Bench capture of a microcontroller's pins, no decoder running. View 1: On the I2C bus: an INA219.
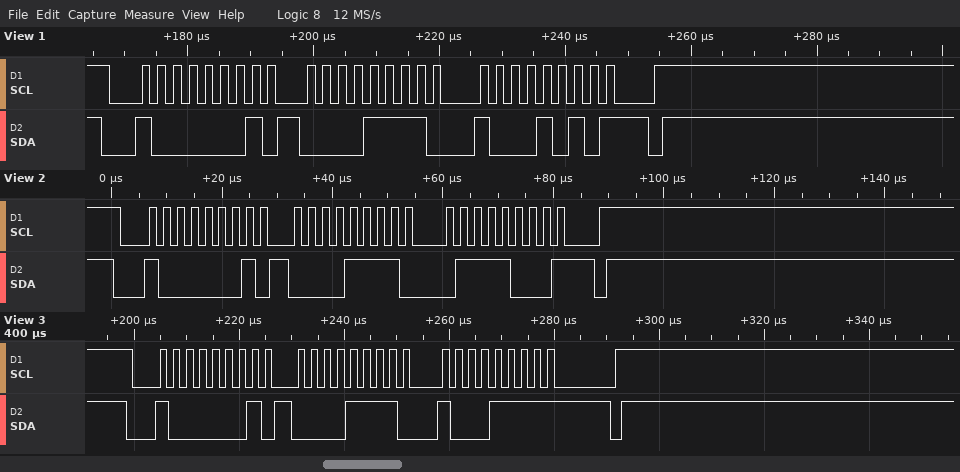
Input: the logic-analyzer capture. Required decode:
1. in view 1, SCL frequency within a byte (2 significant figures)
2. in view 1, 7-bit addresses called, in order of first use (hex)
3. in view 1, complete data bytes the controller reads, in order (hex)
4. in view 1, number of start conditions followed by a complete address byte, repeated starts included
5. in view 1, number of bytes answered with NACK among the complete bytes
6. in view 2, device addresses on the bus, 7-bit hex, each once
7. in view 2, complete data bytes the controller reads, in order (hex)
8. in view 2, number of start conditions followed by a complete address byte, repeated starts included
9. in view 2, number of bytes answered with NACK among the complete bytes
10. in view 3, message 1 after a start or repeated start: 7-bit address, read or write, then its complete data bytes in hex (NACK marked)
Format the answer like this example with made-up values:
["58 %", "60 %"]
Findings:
["400 kHz", "0x40", "0F 8A", "1", "1", "0x40", "0F 78", "1", "1", "0x40 read: 0F 8F NACK"]
